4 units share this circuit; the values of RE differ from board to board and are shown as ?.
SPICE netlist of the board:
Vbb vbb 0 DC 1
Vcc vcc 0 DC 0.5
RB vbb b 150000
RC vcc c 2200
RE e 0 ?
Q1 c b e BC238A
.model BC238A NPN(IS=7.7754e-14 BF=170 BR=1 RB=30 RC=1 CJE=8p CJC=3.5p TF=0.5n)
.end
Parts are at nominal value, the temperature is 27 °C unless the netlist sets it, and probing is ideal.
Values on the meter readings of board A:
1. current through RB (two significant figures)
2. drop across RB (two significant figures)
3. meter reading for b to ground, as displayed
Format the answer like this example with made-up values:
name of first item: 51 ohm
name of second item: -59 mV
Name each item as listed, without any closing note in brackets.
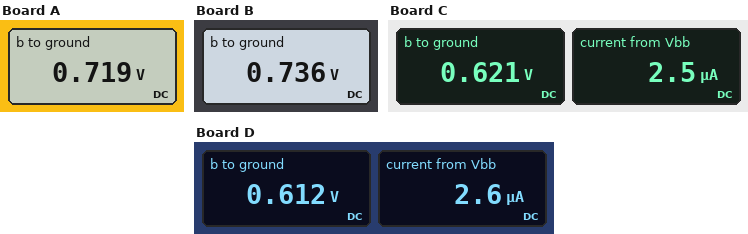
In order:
current through RB: 1.9 µA
drop across RB: 280 mV
meter reading for b to ground, as displayed: 0.719 V
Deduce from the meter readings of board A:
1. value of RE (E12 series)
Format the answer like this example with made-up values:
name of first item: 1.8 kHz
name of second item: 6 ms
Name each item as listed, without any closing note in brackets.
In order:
value of RE: 1.8 kΩ
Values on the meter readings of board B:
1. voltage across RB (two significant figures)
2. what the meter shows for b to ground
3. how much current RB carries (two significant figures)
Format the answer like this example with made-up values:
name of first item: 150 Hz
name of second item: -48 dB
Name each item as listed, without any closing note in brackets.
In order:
voltage across RB: 260 mV
what the meter shows for b to ground: 0.736 V
how much current RB carries: 1.8 µA
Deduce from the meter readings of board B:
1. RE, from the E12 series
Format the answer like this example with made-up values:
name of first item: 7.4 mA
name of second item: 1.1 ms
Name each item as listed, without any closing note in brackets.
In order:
RE, from the E12 series: 2.2 kΩ
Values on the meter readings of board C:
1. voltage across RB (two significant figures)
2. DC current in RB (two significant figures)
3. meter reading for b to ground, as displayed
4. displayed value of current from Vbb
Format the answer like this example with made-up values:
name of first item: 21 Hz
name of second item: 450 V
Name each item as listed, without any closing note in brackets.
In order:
voltage across RB: 380 mV
DC current in RB: 2.5 µA
meter reading for b to ground, as displayed: 0.621 V
displayed value of current from Vbb: 2.5 µA
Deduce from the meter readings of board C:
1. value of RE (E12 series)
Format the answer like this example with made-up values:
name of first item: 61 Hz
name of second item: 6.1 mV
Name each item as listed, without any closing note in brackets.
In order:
value of RE: 470 Ω
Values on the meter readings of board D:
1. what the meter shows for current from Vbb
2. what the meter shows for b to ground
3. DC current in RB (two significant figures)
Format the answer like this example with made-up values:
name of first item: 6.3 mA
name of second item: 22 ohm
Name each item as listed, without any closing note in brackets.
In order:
what the meter shows for current from Vbb: 2.6 µA
what the meter shows for b to ground: 0.612 V
DC current in RB: 2.6 µA
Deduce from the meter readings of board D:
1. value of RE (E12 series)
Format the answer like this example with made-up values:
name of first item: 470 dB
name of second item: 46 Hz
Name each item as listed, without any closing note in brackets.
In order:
value of RE: 390 Ω
